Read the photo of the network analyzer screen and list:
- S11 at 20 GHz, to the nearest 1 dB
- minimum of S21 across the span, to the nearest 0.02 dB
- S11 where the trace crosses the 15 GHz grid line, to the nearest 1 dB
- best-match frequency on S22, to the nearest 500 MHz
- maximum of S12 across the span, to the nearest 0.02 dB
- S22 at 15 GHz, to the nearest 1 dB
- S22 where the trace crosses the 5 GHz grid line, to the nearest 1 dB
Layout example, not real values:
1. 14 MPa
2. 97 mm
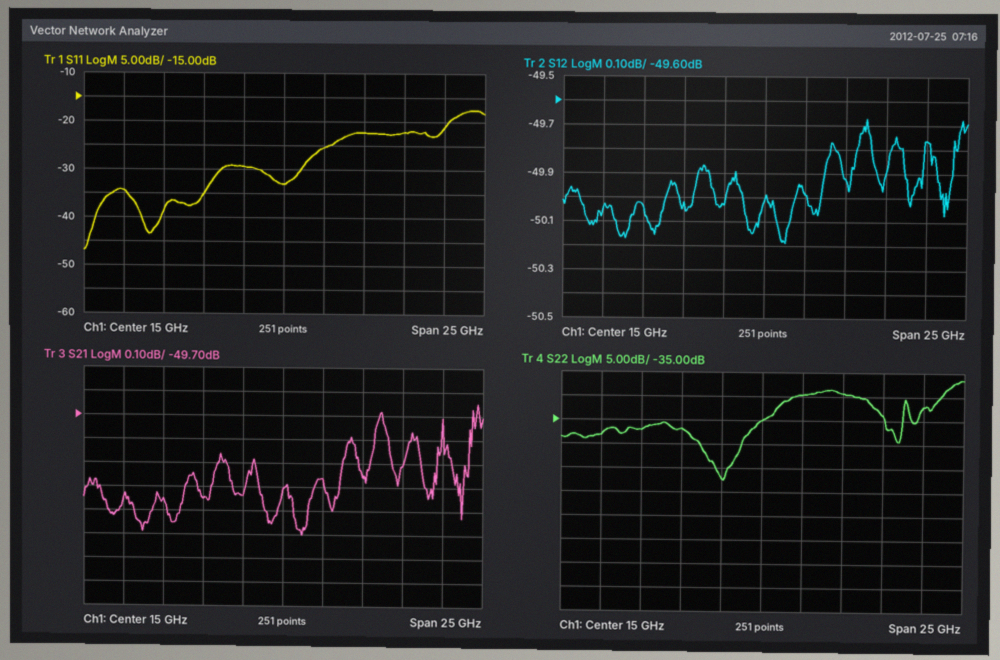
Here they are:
1. -22 dB
2. -50.20 dB
3. -33 dB
4. 12.5 GHz
5. -49.68 dB
6. -35 dB
7. -38 dB
